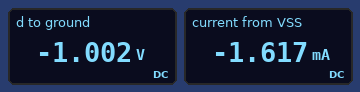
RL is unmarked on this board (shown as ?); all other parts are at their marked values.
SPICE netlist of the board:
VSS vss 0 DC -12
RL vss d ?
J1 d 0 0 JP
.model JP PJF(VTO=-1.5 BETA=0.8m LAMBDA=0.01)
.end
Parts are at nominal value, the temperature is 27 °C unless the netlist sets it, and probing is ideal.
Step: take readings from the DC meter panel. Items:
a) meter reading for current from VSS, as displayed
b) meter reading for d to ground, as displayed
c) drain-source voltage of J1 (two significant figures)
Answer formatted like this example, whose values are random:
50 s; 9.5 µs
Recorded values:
-1.617 mA; -1.002 V; -1.0 V
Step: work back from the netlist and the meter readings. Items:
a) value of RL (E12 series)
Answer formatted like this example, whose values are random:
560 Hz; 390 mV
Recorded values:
6.8 kΩ
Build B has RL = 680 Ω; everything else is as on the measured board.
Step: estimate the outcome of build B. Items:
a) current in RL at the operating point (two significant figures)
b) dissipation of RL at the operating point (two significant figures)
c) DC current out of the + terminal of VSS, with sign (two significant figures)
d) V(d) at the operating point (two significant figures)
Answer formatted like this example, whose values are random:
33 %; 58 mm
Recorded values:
2.0 mA; 2.7 mW; -2.0 mA; -11 V
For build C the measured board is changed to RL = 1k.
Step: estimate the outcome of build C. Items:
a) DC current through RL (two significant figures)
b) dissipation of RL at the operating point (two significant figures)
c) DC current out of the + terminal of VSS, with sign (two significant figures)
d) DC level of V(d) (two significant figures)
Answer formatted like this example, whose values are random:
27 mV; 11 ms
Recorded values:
2.0 mA; 3.9 mW; -2.0 mA; -10 V
